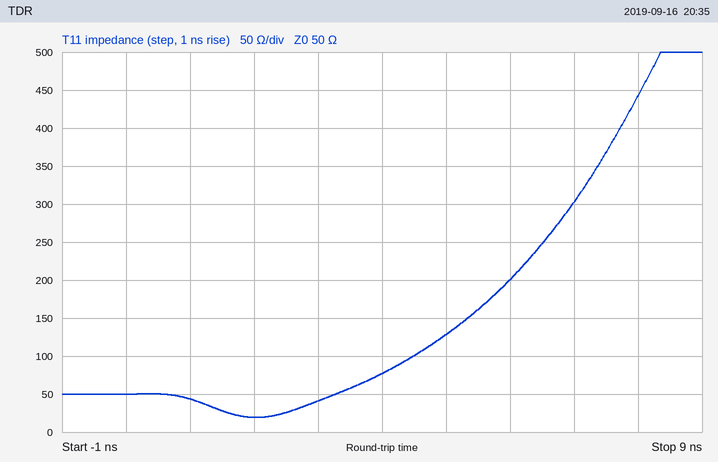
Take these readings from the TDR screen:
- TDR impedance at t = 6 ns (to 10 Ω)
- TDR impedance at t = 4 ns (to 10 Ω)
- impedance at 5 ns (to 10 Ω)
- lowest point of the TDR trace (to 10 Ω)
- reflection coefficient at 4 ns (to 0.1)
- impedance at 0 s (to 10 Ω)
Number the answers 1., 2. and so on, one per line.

1. 200 Ω
2. 80 Ω
3. 130 Ω
4. 20 Ω
5. +0.2
6. 50 Ω
